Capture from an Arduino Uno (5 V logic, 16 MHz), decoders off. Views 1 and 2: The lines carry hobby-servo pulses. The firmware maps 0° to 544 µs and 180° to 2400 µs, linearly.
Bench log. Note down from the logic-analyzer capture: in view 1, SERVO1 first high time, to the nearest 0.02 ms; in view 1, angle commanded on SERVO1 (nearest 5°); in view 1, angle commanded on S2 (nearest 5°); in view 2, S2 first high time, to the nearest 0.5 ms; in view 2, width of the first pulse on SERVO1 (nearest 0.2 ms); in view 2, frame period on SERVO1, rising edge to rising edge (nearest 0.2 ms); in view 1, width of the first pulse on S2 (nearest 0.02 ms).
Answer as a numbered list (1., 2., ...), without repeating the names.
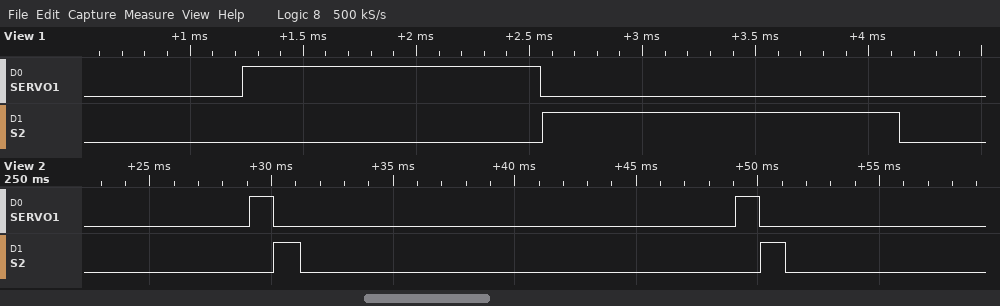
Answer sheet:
1. 1.32 ms
2. 75°
3. 100°
4. 1.0 ms
5. 1.0 ms
6. 20.0 ms
7. 1.58 ms
